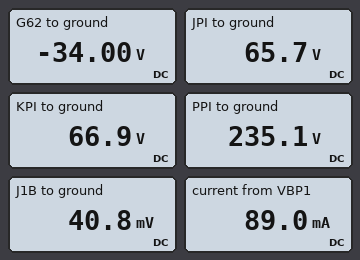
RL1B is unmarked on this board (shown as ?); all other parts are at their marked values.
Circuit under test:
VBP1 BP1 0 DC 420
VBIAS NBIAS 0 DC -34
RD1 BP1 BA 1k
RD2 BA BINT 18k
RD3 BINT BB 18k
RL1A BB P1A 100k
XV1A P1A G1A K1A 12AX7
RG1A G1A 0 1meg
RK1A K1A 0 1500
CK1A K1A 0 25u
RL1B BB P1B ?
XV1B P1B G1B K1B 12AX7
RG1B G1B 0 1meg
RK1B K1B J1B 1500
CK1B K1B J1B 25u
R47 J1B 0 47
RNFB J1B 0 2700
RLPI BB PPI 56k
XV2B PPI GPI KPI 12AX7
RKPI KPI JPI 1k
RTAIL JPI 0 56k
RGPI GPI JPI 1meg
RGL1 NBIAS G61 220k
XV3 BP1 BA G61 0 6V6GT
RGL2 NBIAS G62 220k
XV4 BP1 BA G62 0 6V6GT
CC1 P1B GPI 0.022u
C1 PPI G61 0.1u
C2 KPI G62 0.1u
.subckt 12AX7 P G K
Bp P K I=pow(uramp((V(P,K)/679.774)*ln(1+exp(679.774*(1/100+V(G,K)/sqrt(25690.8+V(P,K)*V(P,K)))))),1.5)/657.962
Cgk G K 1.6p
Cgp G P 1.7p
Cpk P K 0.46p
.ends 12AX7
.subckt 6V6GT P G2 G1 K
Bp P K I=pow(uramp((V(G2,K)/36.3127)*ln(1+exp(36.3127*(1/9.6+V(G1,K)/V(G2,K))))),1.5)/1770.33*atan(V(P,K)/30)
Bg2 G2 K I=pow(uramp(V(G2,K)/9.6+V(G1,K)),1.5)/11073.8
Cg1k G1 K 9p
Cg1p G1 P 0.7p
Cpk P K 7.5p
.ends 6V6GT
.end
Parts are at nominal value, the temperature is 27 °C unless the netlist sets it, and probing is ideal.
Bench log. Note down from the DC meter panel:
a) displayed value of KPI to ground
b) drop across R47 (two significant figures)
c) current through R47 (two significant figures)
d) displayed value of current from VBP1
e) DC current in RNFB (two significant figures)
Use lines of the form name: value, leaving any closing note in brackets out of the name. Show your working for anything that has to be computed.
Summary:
displayed value of KPI to ground: 66.9 V
drop across R47: 40.8 mV = 41 mV
current through R47: (40.8 mV) / 47 Ω = 870 µA
displayed value of current from VBP1: 89.0 mA
DC current in RNFB: (40.8 mV) / 2.7 kΩ = 15 µA
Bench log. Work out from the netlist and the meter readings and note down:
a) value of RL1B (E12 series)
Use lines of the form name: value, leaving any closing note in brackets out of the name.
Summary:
value of RL1B: 150 kΩ
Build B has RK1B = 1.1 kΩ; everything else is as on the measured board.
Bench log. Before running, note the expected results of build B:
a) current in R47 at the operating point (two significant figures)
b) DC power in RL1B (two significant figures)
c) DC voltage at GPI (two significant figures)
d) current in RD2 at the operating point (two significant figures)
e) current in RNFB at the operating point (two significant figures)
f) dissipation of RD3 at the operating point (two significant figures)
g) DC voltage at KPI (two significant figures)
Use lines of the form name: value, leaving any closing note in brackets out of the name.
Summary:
current in R47 at the operating point: 960 µA
DC power in RL1B: 140 mW
DC voltage at GPI: 65 V
current in RD2 at the operating point: 3.2 mA
current in RNFB at the operating point: 17 µA
dissipation of RD3 at the operating point: 180 mW
DC voltage at KPI: 66 V
